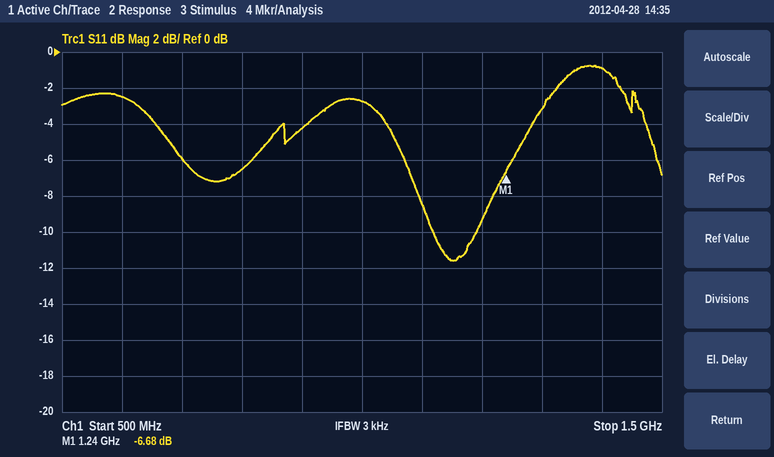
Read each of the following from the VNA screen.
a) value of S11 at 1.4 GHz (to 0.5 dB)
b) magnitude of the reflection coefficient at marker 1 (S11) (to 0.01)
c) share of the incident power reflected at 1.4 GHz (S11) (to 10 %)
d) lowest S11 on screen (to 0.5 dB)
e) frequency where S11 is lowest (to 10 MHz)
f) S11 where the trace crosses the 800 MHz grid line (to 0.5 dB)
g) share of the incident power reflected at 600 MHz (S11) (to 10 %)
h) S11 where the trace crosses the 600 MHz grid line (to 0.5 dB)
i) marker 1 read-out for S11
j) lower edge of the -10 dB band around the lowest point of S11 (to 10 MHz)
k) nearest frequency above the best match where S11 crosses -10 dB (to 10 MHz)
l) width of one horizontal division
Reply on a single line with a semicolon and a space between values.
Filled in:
-1.0 dB; 0.46; 80 %; -11.5 dB; 1.15 GHz; -6.5 dB; 60 %; -2.5 dB; -6.68 dB; 1.12 GHz; 1.19 GHz; 100 MHz
